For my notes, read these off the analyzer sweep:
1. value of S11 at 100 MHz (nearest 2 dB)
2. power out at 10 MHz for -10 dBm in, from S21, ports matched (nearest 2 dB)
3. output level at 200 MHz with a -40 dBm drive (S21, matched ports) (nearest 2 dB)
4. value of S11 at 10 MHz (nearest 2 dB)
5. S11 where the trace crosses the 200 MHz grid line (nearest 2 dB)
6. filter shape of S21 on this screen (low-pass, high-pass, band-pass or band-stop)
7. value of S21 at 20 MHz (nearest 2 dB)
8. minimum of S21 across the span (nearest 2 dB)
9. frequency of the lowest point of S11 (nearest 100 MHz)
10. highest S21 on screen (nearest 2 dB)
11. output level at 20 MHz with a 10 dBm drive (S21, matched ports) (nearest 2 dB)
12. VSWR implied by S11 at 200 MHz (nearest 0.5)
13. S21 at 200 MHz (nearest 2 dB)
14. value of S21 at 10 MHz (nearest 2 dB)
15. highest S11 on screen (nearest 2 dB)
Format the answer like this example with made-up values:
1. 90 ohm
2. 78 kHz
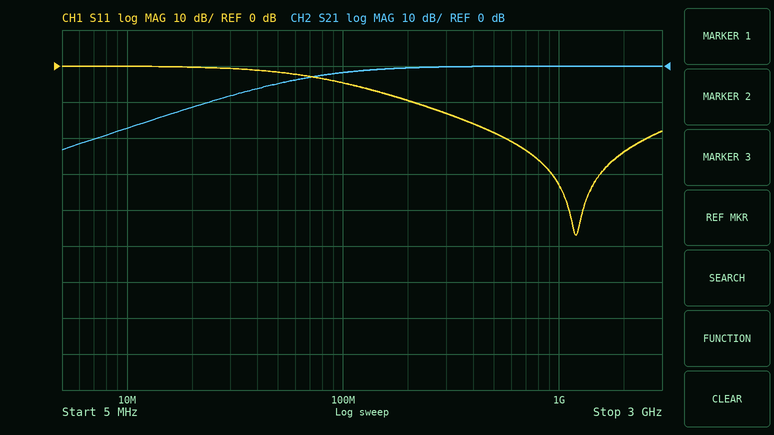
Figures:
1. -4 dB
2. -28 dBm
3. -40 dBm
4. 0 dB
5. -10 dB
6. high-pass
7. -12 dB
8. -24 dB
9. 1.2 GHz
10. 0 dB
11. -2 dBm
12. 2.0
13. 0 dB
14. -18 dB
15. 0 dB
